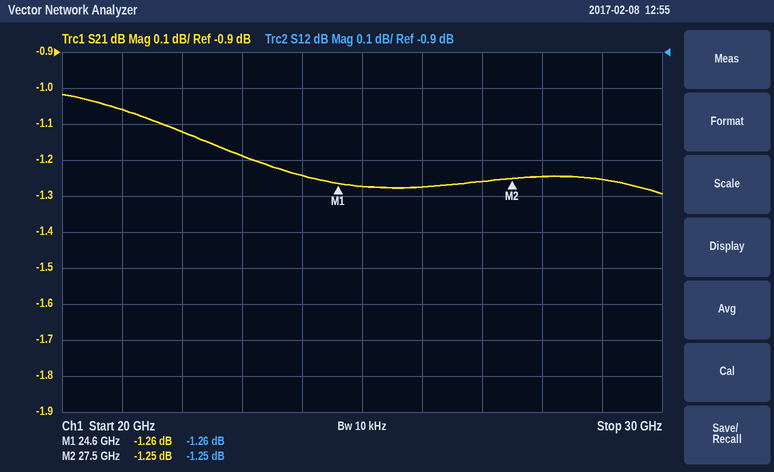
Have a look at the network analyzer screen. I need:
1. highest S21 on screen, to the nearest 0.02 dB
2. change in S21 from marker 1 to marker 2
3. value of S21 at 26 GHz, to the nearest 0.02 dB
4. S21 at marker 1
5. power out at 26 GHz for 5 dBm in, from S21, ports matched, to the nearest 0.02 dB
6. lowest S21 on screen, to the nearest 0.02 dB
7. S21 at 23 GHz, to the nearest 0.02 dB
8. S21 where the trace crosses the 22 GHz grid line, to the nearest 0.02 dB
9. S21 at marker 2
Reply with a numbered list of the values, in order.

1. -1.02 dB
2. 0.01 dB
3. -1.28 dB
4. -1.26 dB
5. 3.72 dBm
6. -1.30 dB
7. -1.18 dB
8. -1.12 dB
9. -1.25 dB
